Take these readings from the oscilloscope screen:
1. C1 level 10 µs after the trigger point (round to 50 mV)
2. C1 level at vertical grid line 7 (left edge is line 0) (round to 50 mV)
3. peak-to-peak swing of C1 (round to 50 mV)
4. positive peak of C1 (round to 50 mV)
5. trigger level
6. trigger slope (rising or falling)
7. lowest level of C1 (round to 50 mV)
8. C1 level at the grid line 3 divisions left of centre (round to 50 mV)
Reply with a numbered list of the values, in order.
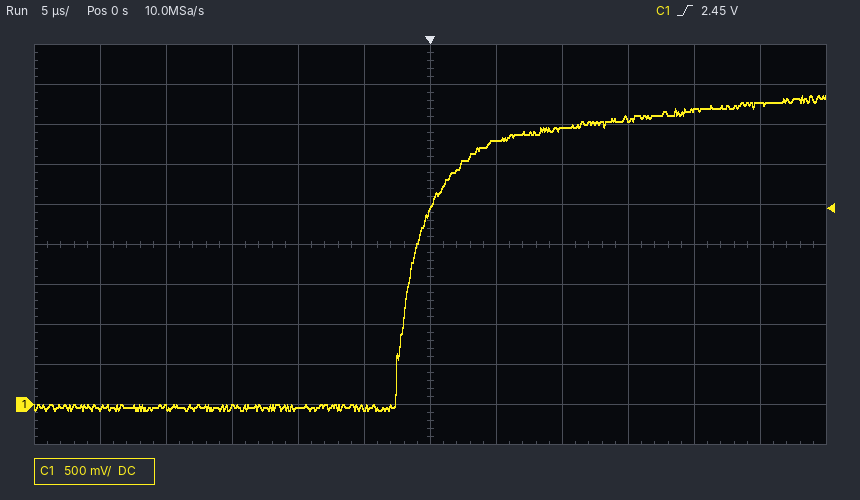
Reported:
1. 3.45 V
2. 3.30 V
3. 3.95 V
4. 3.85 V
5. 2.45 V
6. rising
7. -100 mV
8. -50 mV
